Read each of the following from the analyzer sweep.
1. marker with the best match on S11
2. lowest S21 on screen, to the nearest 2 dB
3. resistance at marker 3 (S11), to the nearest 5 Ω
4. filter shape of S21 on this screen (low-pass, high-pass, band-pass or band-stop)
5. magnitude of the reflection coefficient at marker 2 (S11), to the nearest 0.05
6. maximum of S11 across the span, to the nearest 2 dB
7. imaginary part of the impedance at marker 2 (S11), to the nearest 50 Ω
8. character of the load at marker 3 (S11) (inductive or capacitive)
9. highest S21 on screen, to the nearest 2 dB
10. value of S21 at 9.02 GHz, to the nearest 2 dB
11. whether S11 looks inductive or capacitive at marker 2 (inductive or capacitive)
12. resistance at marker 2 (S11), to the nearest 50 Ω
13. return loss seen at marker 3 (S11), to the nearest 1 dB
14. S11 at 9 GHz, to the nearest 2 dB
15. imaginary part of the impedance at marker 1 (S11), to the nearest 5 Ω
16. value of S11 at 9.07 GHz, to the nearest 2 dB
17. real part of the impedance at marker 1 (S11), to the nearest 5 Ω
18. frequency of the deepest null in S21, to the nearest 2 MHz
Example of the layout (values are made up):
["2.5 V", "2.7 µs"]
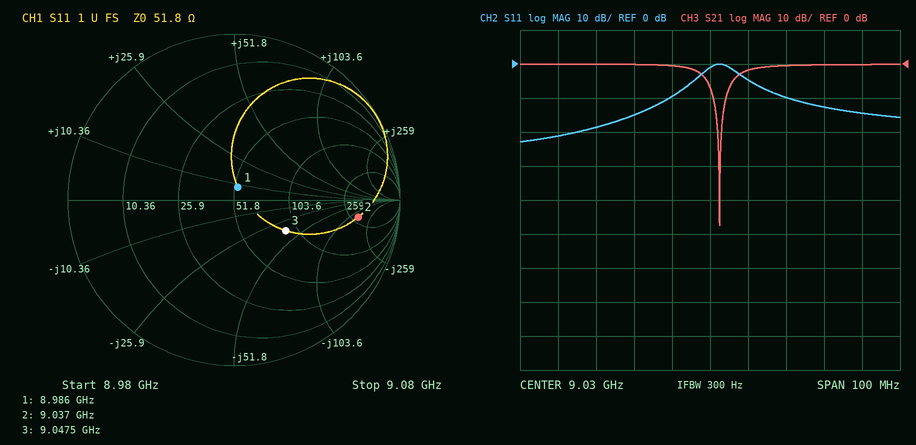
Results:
["marker 1", "-48 dB", "90 Ω", "band-stop", "0.75", "0 dB", "-150 Ω", "capacitive", "0 dB", "0 dB", "capacitive", "300 Ω", "9 dB", "-18 dB", "+10 Ω", "-14 dB", "55 Ω", "9.032 GHz"]
